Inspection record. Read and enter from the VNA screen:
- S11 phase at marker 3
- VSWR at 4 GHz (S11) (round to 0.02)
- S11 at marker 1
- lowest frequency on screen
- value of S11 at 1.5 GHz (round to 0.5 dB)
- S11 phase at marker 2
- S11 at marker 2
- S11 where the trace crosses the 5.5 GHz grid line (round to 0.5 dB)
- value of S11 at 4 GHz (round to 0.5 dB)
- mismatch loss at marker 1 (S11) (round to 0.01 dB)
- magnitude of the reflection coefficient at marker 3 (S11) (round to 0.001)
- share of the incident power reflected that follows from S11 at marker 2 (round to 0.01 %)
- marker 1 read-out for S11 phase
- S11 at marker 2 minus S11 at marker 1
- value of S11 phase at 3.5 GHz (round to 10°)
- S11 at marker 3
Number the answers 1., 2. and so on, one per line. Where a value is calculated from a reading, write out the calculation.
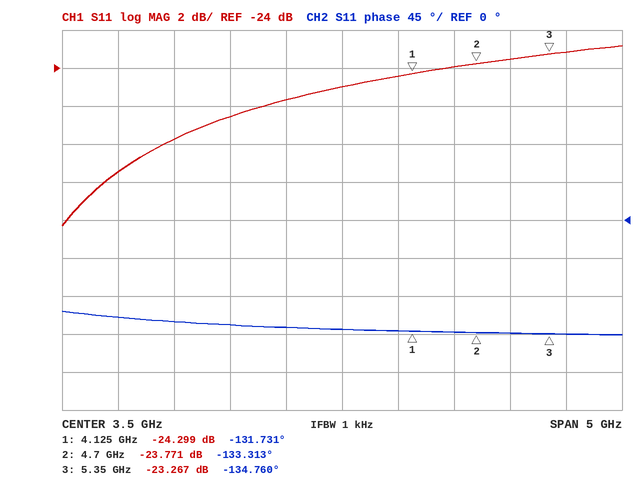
1. -134.760°
2. |Γ| = 10^(-24.5/20) = 0.0596; VSWR = (1 + 0.0596)/(1 − 0.0596) ≈ 1.13, so 1.12 to the nearest 0.02
3. -24.299 dB
4. 1 GHz
5. -29.5 dB
6. -133.313°
7. -23.771 dB
8. -23.0 dB
9. -24.5 dB
10. −10 log10(1 − 10^(-24.299/10)) ≈ 0.02 dB
11. 10^(-23.267/20) ≈ 0.069
12. 10^(-23.771/10) ≈ 0.42 %
13. -131.731°
14. -23.771 − (-24.299) = 0.528 dB
15. -130°
16. -23.267 dB
